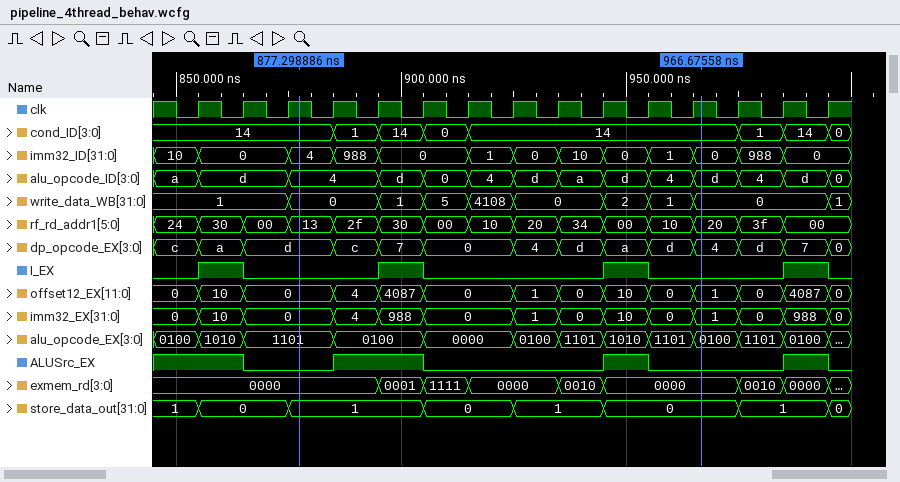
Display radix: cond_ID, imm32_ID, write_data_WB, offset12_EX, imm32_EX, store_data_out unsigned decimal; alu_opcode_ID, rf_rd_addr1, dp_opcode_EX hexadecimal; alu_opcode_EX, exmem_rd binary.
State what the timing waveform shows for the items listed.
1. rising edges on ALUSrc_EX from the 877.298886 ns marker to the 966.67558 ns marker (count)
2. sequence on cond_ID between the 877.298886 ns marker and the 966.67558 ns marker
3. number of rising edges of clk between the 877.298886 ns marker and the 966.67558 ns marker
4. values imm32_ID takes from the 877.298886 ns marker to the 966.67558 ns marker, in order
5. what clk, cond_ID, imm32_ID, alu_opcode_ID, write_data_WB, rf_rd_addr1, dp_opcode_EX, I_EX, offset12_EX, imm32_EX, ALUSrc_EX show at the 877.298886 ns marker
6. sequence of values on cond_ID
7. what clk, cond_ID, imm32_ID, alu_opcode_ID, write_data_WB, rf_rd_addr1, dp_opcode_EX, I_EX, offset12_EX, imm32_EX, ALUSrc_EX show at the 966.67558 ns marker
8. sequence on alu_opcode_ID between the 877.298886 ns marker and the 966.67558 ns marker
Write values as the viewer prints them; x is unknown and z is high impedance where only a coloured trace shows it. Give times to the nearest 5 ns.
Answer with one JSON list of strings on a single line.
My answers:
["2", "14, 1, 14, 0, 14", "9", "4, 988, 0, 1, 0, 10, 0, 1, 0", "clk=1, cond_ID=14, imm32_ID=4, alu_opcode_ID=4, write_data_WB=0, rf_rd_addr1=13, dp_opcode_EX=d, I_EX=0, offset12_EX=0, imm32_EX=0, ALUSrc_EX=0", "14, 1, 14, 0, 14, 1, 14, 0", "clk=1, cond_ID=14, imm32_ID=0, alu_opcode_ID=d, write_data_WB=0, rf_rd_addr1=20, dp_opcode_EX=4, I_EX=0, offset12_EX=1, imm32_EX=1, ALUSrc_EX=0", "4, d, 0, 4, d, a, d, 4, d"]
